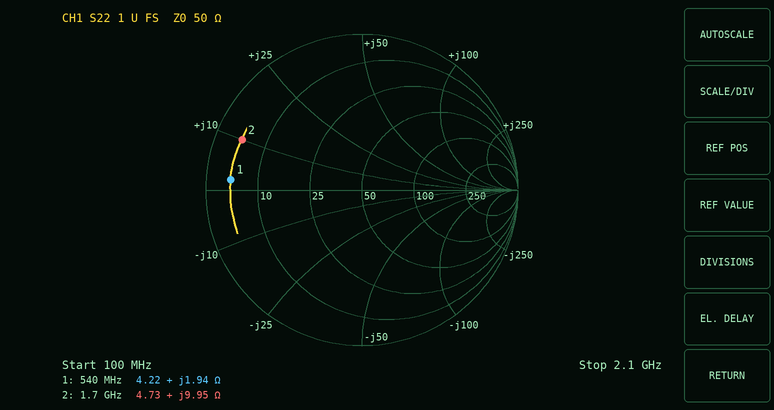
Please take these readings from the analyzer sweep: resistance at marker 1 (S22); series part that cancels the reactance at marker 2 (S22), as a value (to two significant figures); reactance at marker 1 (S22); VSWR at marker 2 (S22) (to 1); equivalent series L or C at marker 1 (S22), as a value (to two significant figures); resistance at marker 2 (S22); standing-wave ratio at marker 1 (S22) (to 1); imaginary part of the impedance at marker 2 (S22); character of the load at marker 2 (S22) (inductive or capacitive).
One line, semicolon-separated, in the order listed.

4.22 Ω; 9.4 pF; +1.94 Ω; 11; 570 pH; 4.73 Ω; 12; +9.95 Ω; inductive
